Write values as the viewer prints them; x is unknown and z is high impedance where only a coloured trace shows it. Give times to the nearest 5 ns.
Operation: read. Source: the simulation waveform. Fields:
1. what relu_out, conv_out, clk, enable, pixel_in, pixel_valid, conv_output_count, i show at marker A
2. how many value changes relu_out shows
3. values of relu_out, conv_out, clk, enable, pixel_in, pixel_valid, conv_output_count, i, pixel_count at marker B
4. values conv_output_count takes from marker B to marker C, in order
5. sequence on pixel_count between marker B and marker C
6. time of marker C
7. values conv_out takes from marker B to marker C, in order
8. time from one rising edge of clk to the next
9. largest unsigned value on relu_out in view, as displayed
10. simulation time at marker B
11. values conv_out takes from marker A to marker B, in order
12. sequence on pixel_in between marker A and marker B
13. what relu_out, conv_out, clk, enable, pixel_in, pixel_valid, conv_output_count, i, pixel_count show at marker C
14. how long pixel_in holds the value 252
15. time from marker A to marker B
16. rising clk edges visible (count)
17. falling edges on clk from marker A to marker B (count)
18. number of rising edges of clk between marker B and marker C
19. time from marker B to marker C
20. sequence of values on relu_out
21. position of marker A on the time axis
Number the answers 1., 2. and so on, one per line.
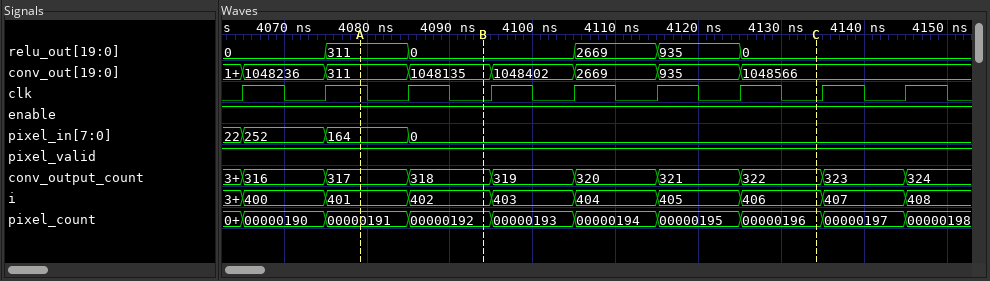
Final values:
1. relu_out=311, conv_out=311, clk=1, enable=1, pixel_in=164, pixel_valid=1, conv_output_count=317, i=401
2. 5
3. relu_out=0, conv_out=1048135, clk=0, enable=1, pixel_in=0, pixel_valid=1, conv_output_count=318, i=402, pixel_count=00000192
4. 318, 319, 320, 321, 322
5. 00000192, 00000193, 00000194, 00000195, 00000196
6. 4135 ns
7. 1048135, 1048402, 2669, 935, 1048566
8. 10 ns
9. 2669
10. 4095 ns
11. 311, 1048135
12. 164, 0
13. relu_out=0, conv_out=1048566, clk=0, enable=1, pixel_in=0, pixel_valid=1, conv_output_count=322, i=406, pixel_count=00000196
14. 10 ns
15. 15 ns
16. 9
17. 2
18. 4
19. 40 ns
20. 0, 311, 0, 2669, 935, 0
21. 4080 ns
